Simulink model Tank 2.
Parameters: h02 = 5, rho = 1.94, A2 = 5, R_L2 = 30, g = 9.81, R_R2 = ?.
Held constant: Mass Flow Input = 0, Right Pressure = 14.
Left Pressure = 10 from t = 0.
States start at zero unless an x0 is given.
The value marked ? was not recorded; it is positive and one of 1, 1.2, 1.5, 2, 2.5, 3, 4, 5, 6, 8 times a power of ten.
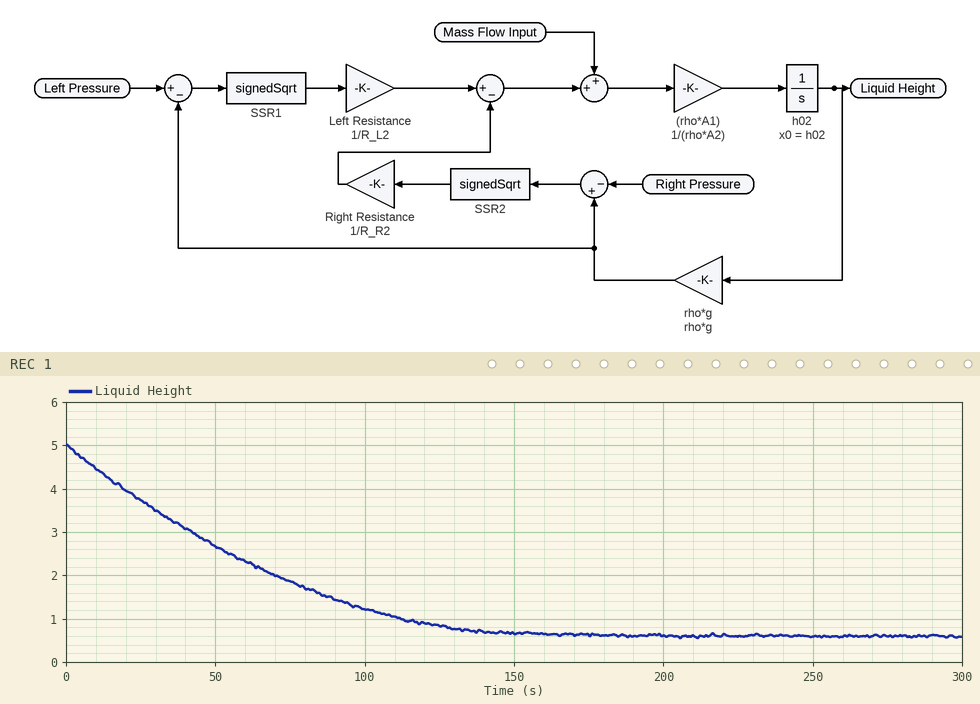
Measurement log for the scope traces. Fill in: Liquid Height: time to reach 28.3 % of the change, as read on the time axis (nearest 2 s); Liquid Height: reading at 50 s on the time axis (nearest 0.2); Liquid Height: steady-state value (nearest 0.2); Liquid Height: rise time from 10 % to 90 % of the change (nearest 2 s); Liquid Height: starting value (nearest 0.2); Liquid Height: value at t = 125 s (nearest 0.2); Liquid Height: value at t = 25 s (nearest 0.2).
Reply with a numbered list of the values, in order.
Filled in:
1. 24 s
2. 2.6
3. 0.6
4. 102 s
5. 5.0
6. 0.8
7. 3.8
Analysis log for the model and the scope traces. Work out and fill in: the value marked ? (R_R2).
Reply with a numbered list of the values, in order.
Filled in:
1. 40
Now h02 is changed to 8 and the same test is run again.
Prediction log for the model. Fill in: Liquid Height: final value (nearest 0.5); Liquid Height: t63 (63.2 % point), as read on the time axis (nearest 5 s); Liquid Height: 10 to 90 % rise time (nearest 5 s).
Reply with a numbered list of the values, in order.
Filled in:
1. 0.5
2. 80 s
3. 130 s
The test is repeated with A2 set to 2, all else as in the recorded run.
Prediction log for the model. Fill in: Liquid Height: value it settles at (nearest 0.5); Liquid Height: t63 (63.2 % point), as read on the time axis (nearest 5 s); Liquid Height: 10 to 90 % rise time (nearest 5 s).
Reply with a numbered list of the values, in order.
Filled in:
1. 0.5
2. 25 s
3. 40 s
